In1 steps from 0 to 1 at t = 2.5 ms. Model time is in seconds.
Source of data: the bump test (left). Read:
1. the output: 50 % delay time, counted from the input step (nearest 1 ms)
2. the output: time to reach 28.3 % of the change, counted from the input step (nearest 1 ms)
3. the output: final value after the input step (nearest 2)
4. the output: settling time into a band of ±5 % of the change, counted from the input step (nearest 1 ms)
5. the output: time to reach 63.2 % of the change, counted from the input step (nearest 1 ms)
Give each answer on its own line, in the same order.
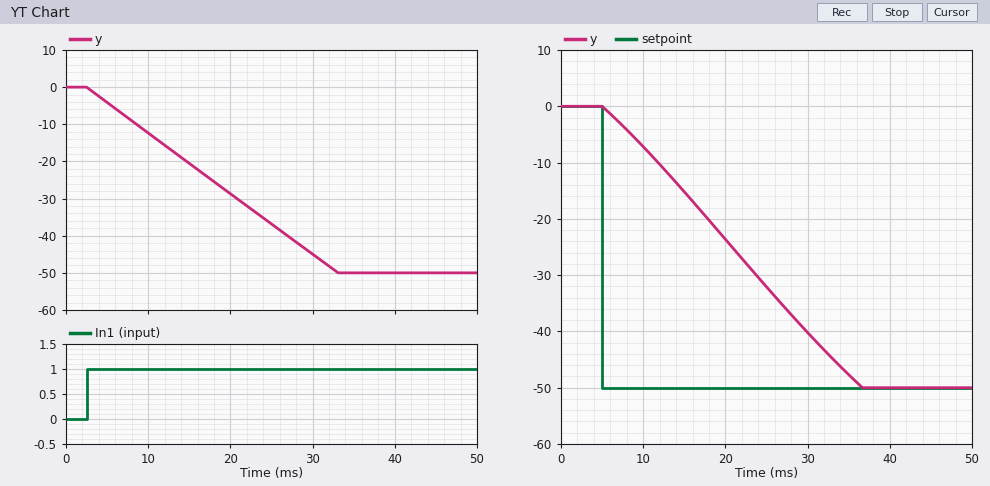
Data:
15 ms
9 ms
-50
29 ms
19 ms
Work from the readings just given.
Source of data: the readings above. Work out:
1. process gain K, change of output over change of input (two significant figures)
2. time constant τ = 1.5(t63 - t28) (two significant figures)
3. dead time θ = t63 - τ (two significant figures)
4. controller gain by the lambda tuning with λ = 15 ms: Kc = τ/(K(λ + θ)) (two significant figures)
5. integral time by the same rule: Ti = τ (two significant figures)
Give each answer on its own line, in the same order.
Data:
-50
15 ms
4.0 ms
-0.016
15 ms
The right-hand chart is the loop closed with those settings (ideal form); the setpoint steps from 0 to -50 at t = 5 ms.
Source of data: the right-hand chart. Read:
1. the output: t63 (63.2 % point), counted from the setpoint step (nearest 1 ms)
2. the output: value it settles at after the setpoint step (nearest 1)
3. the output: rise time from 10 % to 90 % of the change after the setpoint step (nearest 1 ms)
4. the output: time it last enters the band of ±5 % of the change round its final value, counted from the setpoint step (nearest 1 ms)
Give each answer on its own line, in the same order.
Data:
20 ms
-50
25 ms
30 ms
